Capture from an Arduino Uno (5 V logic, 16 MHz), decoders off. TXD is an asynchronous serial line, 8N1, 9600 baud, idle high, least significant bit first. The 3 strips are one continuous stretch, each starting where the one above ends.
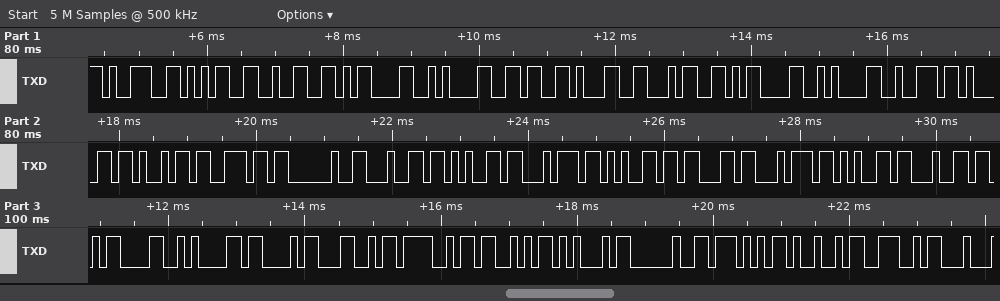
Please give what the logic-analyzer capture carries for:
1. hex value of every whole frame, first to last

39 35 32 0D 0A 36 31 34 0D 0A 72 61 69 6E 20 64 65 74 65 63 74 65 64 0D 0A 43 4C 4F 53 45 20 57 49 4E
